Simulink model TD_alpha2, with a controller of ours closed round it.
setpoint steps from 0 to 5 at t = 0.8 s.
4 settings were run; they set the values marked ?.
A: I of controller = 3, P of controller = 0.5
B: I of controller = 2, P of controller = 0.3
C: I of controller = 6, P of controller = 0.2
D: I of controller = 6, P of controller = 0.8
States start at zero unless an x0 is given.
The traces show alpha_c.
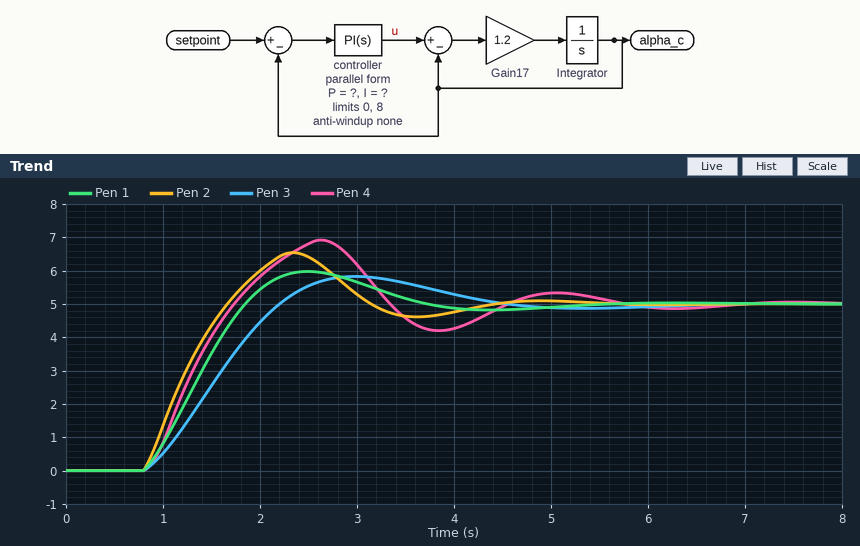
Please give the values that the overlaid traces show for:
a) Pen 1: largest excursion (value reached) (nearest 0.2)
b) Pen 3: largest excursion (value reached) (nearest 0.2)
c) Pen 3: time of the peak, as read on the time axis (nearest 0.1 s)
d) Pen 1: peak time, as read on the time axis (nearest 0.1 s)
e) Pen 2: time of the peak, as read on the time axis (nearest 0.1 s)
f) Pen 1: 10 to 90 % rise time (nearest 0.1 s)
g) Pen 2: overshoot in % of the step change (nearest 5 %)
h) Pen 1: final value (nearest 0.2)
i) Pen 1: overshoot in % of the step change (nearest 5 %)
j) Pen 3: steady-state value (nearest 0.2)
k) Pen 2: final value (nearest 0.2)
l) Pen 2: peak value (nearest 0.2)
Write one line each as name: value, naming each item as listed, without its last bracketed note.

Pen 1: largest excursion (value reached): 6.0
Pen 3: largest excursion (value reached): 5.8
Pen 3: time of the peak, as read on the time axis: 3.0 s
Pen 1: peak time, as read on the time axis: 2.5 s
Pen 2: time of the peak, as read on the time axis: 2.3 s
Pen 1: 10 to 90 % rise time: 0.8 s
Pen 2: overshoot in % of the step change: 30 %
Pen 1: final value: 5.0
Pen 1: overshoot in % of the step change: 20 %
Pen 3: steady-state value: 5.0
Pen 2: final value: 5.0
Pen 2: peak value: 6.6
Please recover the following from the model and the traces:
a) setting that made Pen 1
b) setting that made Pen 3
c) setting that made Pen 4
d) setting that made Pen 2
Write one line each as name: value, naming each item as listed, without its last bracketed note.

setting that made Pen 1: A
setting that made Pen 3: B
setting that made Pen 4: C
setting that made Pen 2: D
